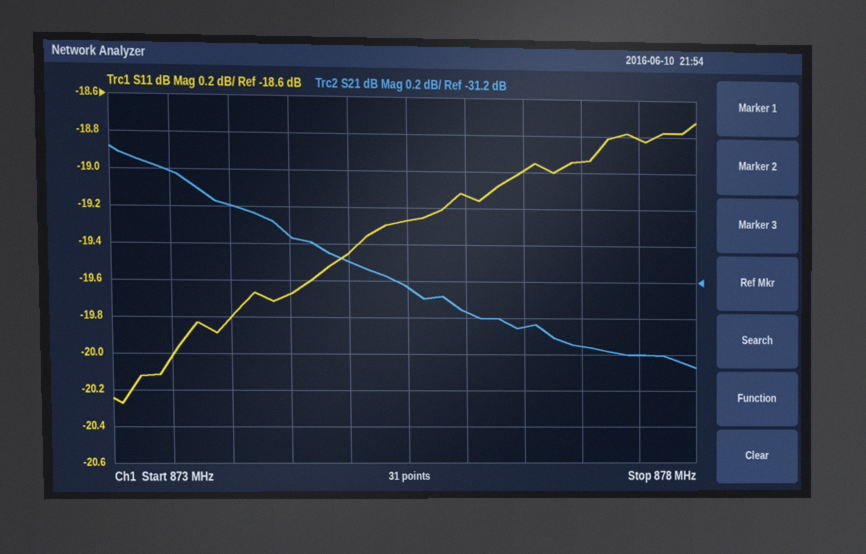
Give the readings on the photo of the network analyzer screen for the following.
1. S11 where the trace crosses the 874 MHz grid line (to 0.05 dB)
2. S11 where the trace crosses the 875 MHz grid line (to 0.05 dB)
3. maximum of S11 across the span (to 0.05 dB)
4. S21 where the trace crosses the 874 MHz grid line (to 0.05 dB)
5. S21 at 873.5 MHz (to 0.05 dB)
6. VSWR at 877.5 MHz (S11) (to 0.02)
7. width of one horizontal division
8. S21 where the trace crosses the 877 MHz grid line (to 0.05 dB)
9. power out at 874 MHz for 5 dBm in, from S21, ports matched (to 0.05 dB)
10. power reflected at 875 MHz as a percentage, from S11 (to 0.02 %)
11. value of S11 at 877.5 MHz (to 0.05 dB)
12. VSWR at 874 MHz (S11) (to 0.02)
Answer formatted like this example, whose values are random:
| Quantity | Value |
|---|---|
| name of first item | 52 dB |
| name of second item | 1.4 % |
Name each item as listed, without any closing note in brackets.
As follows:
| Quantity | Value |
|---|---|
| S11 where the trace crosses the 874 MHz grid line | -19.80 dB |
| S11 where the trace crosses the 875 MHz grid line | -19.45 dB |
| maximum of S11 across the span | -18.70 dB |
| S21 where the trace crosses the 874 MHz grid line | -30.80 dB |
| S21 at 873.5 MHz | -30.60 dB |
| VSWR at 877.5 MHz (S11) | 1.26 |
| width of one horizontal division | 500 kHz |
| S21 where the trace crosses the 877 MHz grid line | -31.55 dB |
| power out at 874 MHz for 5 dBm in, from S21, ports matched | -25.80 dBm |
| power reflected at 875 MHz as a percentage, from S11 | 1.14 % |
| value of S11 at 877.5 MHz | -18.80 dB |
| VSWR at 874 MHz (S11) | 1.22 |
